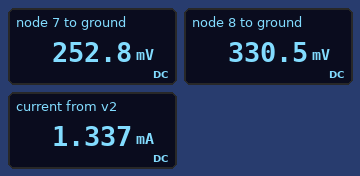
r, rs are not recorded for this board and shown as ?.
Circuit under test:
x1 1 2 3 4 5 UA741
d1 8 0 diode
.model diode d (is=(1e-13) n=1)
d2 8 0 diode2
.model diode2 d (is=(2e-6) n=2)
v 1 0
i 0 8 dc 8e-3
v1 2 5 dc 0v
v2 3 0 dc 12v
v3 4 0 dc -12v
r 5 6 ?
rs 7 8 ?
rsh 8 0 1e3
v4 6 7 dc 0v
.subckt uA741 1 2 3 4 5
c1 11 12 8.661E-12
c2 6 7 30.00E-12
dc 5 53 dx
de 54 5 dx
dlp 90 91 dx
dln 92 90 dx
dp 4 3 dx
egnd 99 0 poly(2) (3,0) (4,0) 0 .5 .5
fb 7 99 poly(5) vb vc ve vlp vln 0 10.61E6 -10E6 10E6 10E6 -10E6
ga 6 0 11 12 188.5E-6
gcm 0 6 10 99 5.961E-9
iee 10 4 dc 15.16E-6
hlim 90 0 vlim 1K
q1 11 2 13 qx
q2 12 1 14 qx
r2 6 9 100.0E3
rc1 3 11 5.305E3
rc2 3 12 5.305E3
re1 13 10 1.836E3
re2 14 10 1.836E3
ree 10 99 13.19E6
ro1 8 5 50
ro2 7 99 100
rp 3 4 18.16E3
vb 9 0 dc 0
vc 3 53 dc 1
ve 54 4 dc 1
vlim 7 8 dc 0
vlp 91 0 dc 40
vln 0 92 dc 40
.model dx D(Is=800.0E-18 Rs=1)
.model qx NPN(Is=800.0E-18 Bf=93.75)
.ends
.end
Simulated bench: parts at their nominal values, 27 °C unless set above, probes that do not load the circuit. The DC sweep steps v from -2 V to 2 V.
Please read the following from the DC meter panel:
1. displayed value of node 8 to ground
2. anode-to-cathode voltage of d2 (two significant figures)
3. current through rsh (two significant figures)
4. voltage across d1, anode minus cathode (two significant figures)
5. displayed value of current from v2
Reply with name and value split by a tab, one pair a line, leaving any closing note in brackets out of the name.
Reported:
displayed value of node 8 to ground	330.5 mV
anode-to-cathode voltage of d2	330 mV
current through rsh	330 µA
voltage across d1, anode minus cathode	330 mV
displayed value of current from v2	1.337 mA
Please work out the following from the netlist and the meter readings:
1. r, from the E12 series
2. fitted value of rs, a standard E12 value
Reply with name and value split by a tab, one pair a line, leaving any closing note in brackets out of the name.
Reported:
r, from the E12 series	39 Ω
fitted value of rs, a standard E12 value	12 Ω
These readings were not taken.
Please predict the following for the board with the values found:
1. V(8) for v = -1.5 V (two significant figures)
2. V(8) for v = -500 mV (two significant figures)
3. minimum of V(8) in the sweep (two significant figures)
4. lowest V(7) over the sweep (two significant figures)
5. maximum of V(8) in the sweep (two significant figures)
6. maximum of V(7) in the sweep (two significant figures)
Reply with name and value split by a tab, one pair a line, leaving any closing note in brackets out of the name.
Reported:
V(8) for v = -1.5 V	-1.0 V
V(8) for v = -500 mV	-87 mV
minimum of V(8) in the sweep	-1.5 V
lowest V(7) over the sweep	-1.6 V
maximum of V(8) in the sweep	510 mV
maximum of V(7) in the sweep	860 mV
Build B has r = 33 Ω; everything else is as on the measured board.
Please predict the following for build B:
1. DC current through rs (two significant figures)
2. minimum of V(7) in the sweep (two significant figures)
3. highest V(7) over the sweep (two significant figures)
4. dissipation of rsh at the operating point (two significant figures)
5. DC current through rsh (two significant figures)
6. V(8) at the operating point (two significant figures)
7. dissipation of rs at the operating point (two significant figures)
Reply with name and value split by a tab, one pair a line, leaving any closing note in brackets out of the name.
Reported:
DC current through rs	6.9 mA
minimum of V(7) in the sweep	-1.7 V
highest V(7) over the sweep	910 mV
dissipation of rsh at the operating point	96 µW
DC current through rsh	310 µA
V(8) at the operating point	310 mV
dissipation of rs at the operating point	570 µW
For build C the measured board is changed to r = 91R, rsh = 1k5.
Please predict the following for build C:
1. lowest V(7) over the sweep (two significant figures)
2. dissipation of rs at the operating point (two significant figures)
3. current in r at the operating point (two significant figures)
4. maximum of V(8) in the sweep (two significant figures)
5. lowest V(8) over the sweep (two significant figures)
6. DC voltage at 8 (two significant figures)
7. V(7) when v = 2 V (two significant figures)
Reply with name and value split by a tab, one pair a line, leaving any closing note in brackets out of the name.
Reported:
lowest V(7) over the sweep	-1.2 V
dissipation of rs at the operating point	170 µW
current in r at the operating point	3.8 mA
maximum of V(8) in the sweep	480 mV
lowest V(8) over the sweep	-1.1 V
DC voltage at 8	390 mV
V(7) when v = 2 V	660 mV
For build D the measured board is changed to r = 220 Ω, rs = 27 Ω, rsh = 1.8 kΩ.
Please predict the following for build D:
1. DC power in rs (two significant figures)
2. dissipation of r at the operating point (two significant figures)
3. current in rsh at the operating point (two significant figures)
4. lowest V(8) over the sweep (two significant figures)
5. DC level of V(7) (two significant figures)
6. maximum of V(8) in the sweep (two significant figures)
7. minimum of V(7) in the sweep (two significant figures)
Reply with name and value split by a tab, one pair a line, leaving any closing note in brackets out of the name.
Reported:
DC power in rs	76 µW
dissipation of r at the operating point	620 µW
current in rsh at the operating point	230 µA
lowest V(8) over the sweep	-21 mV
DC level of V(7)	370 mV
maximum of V(8) in the sweep	460 mV
minimum of V(7) in the sweep	-240 mV
